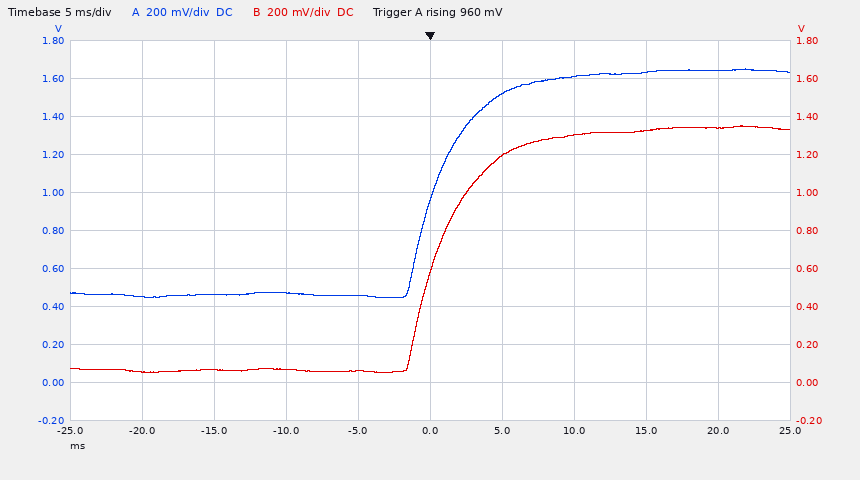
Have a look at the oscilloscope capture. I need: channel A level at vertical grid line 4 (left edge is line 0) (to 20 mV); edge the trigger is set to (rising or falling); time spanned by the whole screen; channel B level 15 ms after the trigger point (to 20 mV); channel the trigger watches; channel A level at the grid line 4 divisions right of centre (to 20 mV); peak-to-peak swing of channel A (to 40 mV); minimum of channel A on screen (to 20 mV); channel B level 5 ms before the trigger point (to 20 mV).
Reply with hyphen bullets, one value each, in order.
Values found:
- 460 mV
- rising
- 50 ms
- 1.32 V
- channel A
- 1.64 V
- 1.20 V
- 440 mV
- 60 mV
